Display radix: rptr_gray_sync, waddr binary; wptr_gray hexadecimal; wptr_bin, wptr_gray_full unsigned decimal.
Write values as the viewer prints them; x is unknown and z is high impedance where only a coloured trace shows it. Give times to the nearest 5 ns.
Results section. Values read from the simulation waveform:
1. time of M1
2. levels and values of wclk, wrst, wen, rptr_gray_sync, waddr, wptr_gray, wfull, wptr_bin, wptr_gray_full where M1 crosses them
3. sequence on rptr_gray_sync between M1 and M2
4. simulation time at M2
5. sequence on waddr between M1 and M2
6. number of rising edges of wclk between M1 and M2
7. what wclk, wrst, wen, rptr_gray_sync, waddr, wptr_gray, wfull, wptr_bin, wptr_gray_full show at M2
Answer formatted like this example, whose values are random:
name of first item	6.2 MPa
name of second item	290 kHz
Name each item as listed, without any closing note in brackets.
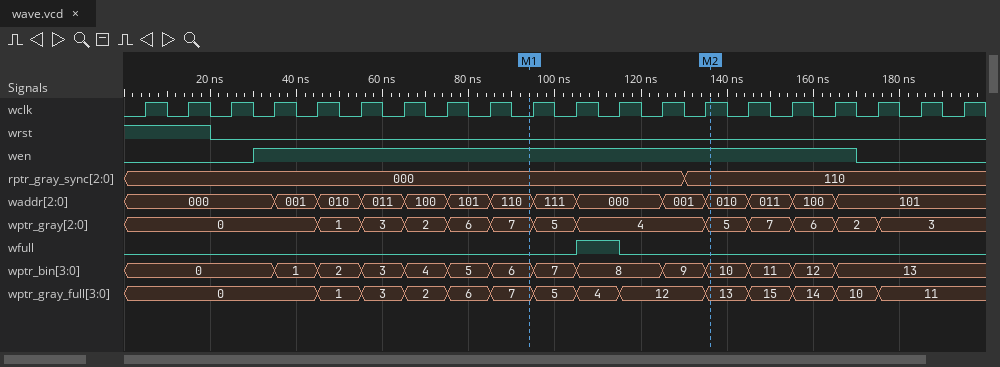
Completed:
time of M1	95 ns
levels and values of wclk, wrst, wen, rptr_gray_sync, waddr, wptr_gray, wfull, wptr_bin, wptr_gray_full where M1 crosses them	wclk=0, wrst=0, wen=1, rptr_gray_sync=000, waddr=110, wptr_gray=7, wfull=0, wptr_bin=6, wptr_gray_full=7
sequence on rptr_gray_sync between M1 and M2	000, 110
simulation time at M2	135 ns
sequence on waddr between M1 and M2	110, 111, 000, 001, 010
number of rising edges of wclk between M1 and M2	5
what wclk, wrst, wen, rptr_gray_sync, waddr, wptr_gray, wfull, wptr_bin, wptr_gray_full show at M2	wclk=1, wrst=0, wen=1, rptr_gray_sync=110, waddr=010, wptr_gray=5, wfull=0, wptr_bin=10, wptr_gray_full=13
